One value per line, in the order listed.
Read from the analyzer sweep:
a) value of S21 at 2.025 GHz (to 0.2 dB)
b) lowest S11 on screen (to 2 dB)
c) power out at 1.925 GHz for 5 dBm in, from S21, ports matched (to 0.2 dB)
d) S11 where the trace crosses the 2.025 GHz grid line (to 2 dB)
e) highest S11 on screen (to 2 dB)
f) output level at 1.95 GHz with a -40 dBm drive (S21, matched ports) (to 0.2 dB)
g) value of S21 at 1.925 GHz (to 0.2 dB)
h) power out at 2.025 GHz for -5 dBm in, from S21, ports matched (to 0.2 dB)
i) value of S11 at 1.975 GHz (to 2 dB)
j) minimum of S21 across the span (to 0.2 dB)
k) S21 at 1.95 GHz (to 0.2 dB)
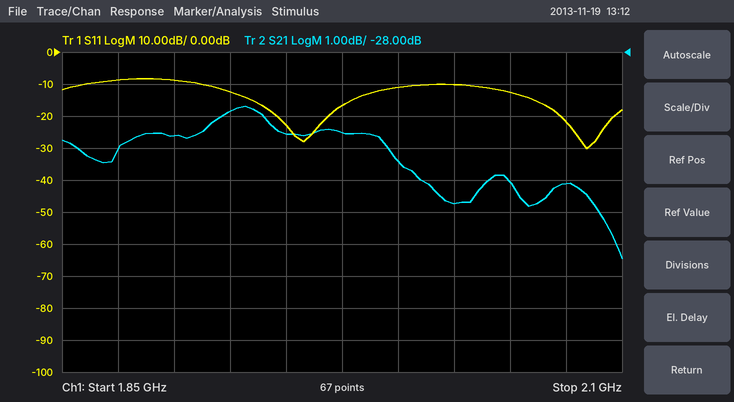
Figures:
-32.8 dB
-30 dB
-24.8 dBm
-10 dB
-8 dB
-70.6 dBm
-29.8 dB
-37.8 dBm
-16 dB
-34.4 dB
-30.6 dB
